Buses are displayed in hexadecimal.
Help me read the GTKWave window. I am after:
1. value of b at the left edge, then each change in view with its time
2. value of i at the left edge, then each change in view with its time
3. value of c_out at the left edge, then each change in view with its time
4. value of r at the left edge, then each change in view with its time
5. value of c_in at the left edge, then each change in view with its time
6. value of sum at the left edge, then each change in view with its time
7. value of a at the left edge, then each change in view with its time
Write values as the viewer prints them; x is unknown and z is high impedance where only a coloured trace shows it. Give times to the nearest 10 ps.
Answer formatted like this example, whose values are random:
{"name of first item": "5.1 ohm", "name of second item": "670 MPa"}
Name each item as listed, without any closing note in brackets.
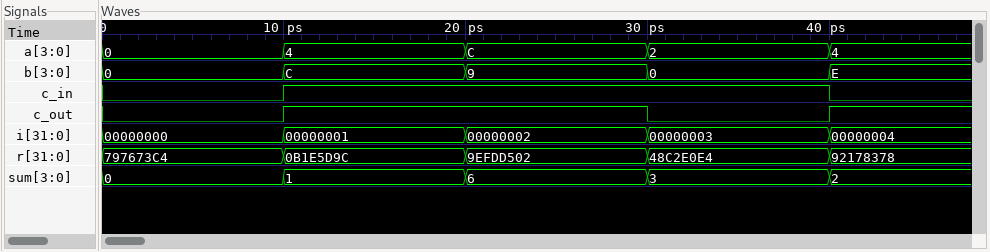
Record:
{"value of b at the left edge, then each change in view with its time": "0, C at 10 ps, 9 at 20 ps, 0 at 30 ps, E at 40 ps", "value of i at the left edge, then each change in view with its time": "00000000, 00000001 at 10 ps, 00000002 at 20 ps, 00000003 at 30 ps, 00000004 at 40 ps", "value of c_out at the left edge, then each change in view with its time": "0, 1 at 10 ps, 0 at 30 ps, 1 at 40 ps", "value of r at the left edge, then each change in view with its time": "797673C4, 0B1E5D9C at 10 ps, 9EFDD502 at 20 ps, 48C2E0E4 at 30 ps, 92178378 at 40 ps", "value of c_in at the left edge, then each change in view with its time": "0, 1 at 10 ps, 0 at 40 ps", "value of sum at the left edge, then each change in view with its time": "0, 1 at 10 ps, 6 at 20 ps, 3 at 30 ps, 2 at 40 ps", "value of a at the left edge, then each change in view with its time": "0, 4 at 10 ps, C at 20 ps, 2 at 30 ps, 4 at 40 ps"}
